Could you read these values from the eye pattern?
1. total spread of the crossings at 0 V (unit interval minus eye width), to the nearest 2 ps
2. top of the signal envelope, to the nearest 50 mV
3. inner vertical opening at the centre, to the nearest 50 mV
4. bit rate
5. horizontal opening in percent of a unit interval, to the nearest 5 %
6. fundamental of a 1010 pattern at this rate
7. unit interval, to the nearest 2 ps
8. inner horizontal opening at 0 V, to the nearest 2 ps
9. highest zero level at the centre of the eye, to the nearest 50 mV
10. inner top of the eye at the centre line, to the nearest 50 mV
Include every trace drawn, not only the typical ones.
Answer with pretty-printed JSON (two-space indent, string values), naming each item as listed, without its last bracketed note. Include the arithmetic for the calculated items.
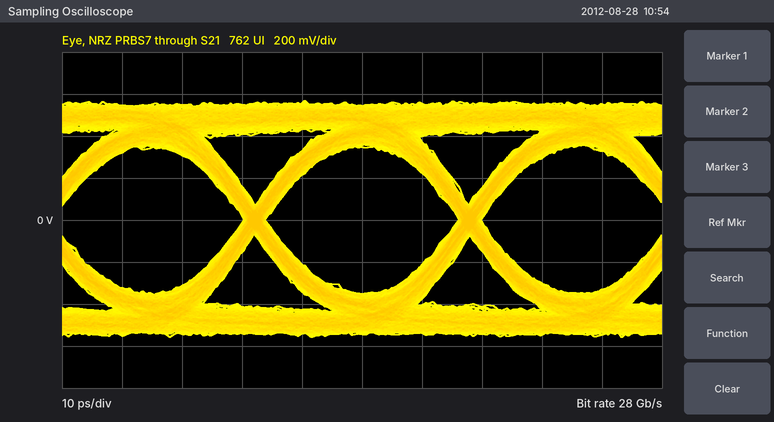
{
  "total spread of the crossings at 0 V (unit interval minus eye width), to the nearest 2 ps": "4 ps",
  "top of the signal envelope, to the nearest 50 mV": "550 mV",
  "inner vertical opening at the centre, to the nearest 50 mV": "700 mV",
  "bit rate": "28 Gb/s",
  "horizontal opening in percent of a unit interval, to the nearest 5 %": "32 ps / 36 ps ≈ 88.9 %, so 90 % to the nearest 5 %",
  "fundamental of a 1010 pattern at this rate": "14 GHz",
  "unit interval, to the nearest 2 ps": "36 ps",
  "inner horizontal opening at 0 V, to the nearest 2 ps": "32 ps",
  "highest zero level at the centre of the eye, to the nearest 50 mV": "-350 mV",
  "inner top of the eye at the centre line, to the nearest 50 mV": "350 mV"
}
